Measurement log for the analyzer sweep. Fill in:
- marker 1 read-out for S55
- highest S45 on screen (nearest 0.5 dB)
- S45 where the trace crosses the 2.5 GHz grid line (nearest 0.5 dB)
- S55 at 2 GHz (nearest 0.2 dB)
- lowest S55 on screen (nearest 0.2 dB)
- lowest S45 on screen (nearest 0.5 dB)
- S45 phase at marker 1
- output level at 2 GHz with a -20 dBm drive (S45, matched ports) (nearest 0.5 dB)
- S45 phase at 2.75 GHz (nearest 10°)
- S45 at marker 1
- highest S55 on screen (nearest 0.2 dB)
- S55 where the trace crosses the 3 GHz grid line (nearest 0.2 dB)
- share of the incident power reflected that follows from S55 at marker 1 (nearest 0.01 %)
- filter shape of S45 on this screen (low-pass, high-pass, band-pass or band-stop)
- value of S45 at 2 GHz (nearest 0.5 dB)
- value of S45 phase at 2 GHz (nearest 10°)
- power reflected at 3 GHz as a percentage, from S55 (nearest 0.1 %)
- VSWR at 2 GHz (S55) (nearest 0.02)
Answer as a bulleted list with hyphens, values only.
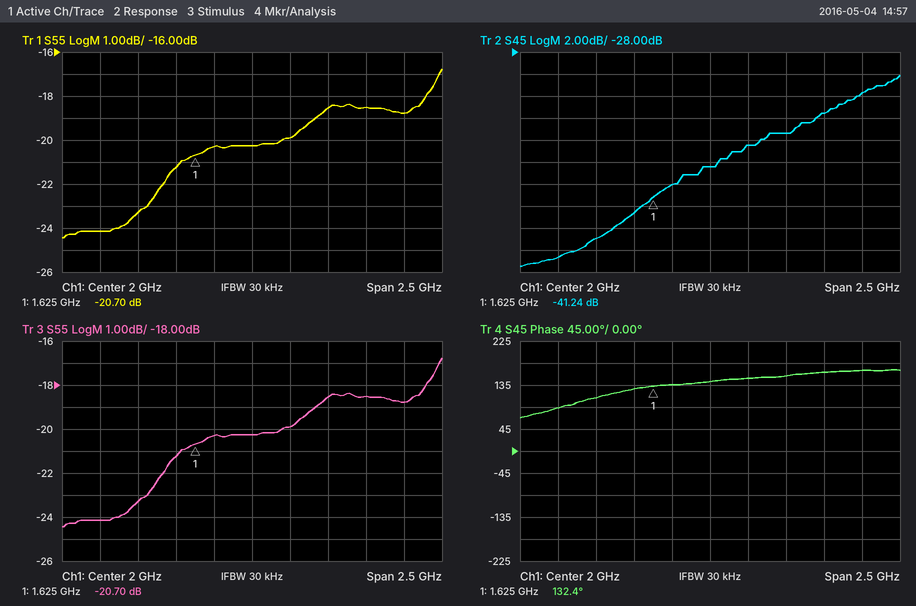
- -20.70 dB
- -30.0 dB
- -35.5 dB
- -20.2 dB
- -24.4 dB
- -47.5 dB
- 132.4°
- -58.5 dBm
- 160°
- -41.24 dB
- -16.8 dB
- -18.8 dB
- 0.85 %
- high-pass
- -38.5 dB
- 140°
- 1.3 %
- 1.22
